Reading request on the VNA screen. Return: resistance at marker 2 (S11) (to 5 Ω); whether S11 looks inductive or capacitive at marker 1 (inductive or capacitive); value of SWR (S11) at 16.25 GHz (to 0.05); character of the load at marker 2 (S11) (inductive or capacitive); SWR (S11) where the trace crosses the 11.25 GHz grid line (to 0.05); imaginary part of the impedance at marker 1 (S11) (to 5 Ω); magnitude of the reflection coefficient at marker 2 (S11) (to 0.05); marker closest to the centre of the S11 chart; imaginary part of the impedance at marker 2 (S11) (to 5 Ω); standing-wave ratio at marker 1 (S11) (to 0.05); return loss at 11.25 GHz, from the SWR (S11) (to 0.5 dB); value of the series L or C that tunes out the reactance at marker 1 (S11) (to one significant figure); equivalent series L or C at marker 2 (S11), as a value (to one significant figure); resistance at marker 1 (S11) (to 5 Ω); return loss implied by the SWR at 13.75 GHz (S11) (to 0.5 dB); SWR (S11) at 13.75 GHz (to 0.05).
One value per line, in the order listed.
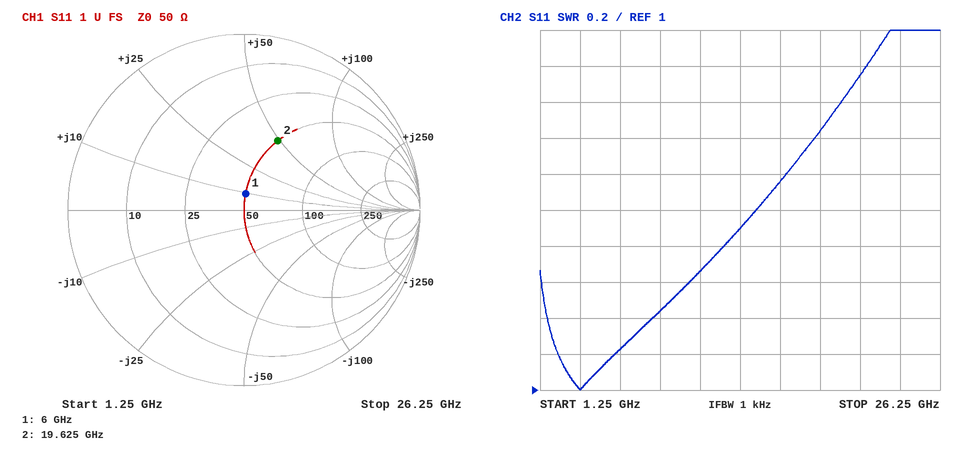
50 Ω
inductive
2.15
inductive
1.65
+10 Ω
0.45
marker 1
+50 Ω
1.20
12.0 dB
3 pF
400 pH
50 Ω
10.0 dB
1.90
